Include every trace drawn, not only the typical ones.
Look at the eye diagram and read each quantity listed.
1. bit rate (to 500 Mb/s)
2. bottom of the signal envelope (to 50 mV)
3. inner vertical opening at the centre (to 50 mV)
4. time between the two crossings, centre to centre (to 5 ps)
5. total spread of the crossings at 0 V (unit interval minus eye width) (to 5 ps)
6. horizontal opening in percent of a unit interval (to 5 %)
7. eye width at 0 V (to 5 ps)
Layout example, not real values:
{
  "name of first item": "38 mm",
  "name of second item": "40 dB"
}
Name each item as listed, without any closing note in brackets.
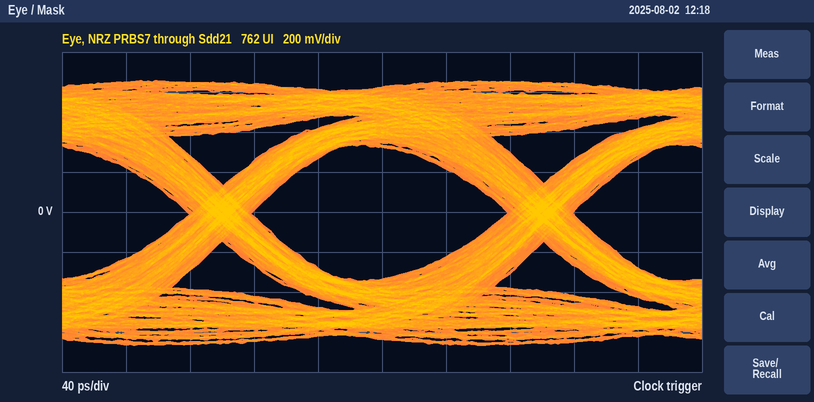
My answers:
{
  "bit rate": "5.0 Gb/s",
  "bottom of the signal envelope": "-650 mV",
  "inner vertical opening at the centre": "650 mV",
  "time between the two crossings, centre to centre": "200 ps",
  "total spread of the crossings at 0 V (unit interval minus eye width)": "40 ps",
  "horizontal opening in percent of a unit interval": "80 %",
  "eye width at 0 V": "160 ps"
}
